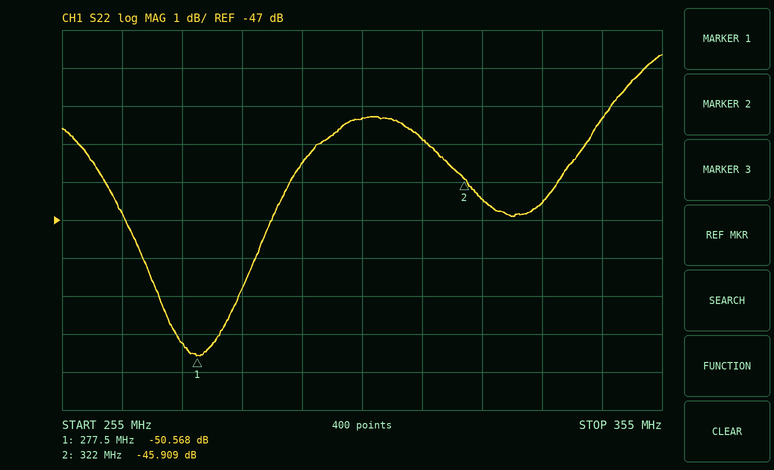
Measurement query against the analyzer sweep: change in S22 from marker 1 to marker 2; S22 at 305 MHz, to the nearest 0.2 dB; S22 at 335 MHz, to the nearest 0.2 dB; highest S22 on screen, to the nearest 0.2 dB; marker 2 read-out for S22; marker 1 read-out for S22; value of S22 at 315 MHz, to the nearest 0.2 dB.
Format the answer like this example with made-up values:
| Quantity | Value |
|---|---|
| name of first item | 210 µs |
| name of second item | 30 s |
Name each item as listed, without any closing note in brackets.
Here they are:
| Quantity | Value |
|---|---|
| change in S22 from marker 1 to marker 2 | 4.659 dB |
| S22 at 305 MHz, to the nearest 0.2 dB | -44.4 dB |
| S22 at 335 MHz, to the nearest 0.2 dB | -46.6 dB |
| highest S22 on screen, to the nearest 0.2 dB | -42.6 dB |
| marker 2 read-out for S22 | -45.909 dB |
| marker 1 read-out for S22 | -50.568 dB |
| value of S22 at 315 MHz, to the nearest 0.2 dB | -44.8 dB |
